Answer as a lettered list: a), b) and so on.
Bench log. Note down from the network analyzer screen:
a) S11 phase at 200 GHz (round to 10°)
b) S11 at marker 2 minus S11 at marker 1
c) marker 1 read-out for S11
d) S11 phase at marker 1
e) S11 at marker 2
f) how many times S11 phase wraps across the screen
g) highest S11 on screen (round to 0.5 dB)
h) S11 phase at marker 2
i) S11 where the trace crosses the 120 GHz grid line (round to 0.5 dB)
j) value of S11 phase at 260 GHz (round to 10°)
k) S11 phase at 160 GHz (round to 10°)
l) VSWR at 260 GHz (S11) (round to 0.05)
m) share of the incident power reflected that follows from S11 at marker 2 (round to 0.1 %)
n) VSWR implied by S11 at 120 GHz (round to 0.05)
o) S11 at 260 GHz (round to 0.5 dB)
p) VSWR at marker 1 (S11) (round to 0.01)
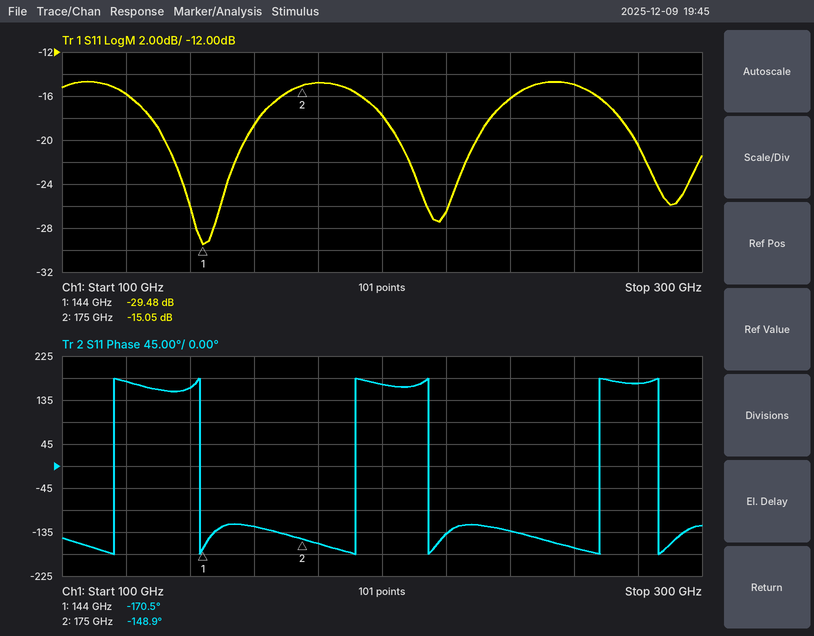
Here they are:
a) 170°
b) 14.43 dB
c) -29.48 dB
d) -170.5°
e) -15.05 dB
f) 6
g) -14.5 dB
h) -148.9°
i) -16.0 dB
j) -170°
k) -120°
l) 1.45
m) 3.1 %
n) 1.40
o) -15.0 dB
p) 1.07
